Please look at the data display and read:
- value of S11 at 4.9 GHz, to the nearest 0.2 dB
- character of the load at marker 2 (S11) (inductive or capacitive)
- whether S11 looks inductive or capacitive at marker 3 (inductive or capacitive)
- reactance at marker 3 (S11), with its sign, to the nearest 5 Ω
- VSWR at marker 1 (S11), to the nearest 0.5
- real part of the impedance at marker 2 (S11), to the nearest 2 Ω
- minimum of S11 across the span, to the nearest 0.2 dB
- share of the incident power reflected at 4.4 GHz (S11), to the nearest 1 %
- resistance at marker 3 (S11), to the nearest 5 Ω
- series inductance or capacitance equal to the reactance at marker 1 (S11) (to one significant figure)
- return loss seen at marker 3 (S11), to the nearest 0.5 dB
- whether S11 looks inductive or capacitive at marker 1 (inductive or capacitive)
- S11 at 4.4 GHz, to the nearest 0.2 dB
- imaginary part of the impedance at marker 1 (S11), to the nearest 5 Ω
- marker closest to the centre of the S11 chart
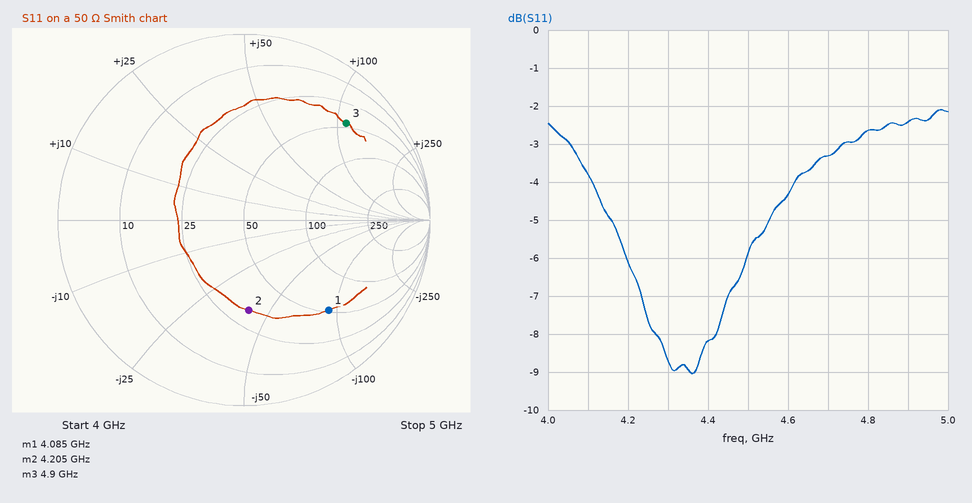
-2.4 dB
capacitive
inductive
+110 Ω
5.0
32 Ω
-9.0 dB
15 %
45 Ω
400 fF
2.5 dB
capacitive
-8.2 dB
-90 Ω
marker 2
